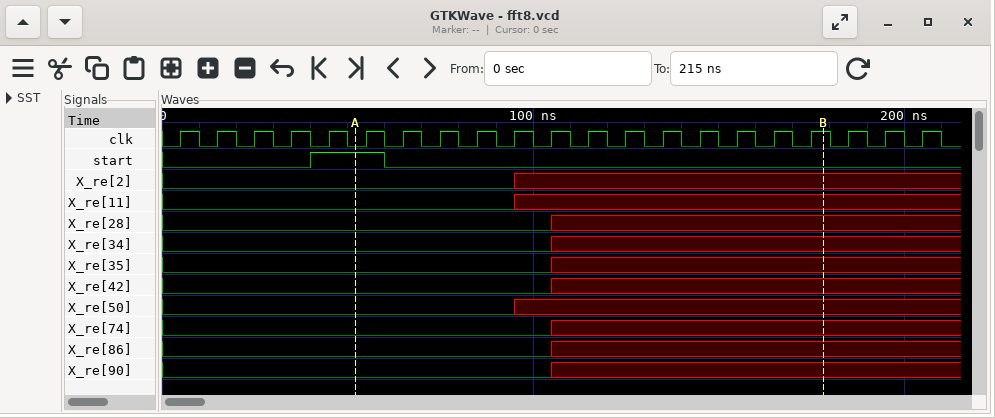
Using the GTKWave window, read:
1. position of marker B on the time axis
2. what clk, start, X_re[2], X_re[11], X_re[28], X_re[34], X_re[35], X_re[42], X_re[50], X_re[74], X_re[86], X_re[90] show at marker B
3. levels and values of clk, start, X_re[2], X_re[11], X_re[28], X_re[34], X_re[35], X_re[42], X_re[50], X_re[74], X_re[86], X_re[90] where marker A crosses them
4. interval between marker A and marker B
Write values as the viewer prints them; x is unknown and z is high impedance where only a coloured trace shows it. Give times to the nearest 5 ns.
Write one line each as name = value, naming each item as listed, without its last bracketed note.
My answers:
position of marker B on the time axis = 180 ns
what clk, start, X_re[2], X_re[11], X_re[28], X_re[34], X_re[35], X_re[42], X_re[50], X_re[74], X_re[86], X_re[90] show at marker B = clk=1, start=0, X_re[2]=x, X_re[11]=x, X_re[28]=x, X_re[34]=x, X_re[35]=x, X_re[42]=x, X_re[50]=x, X_re[74]=x, X_re[86]=x, X_re[90]=x
levels and values of clk, start, X_re[2], X_re[11], X_re[28], X_re[34], X_re[35], X_re[42], X_re[50], X_re[74], X_re[86], X_re[90] where marker A crosses them = clk=0, start=1, X_re[2]=0, X_re[11]=0, X_re[28]=0, X_re[34]=0, X_re[35]=0, X_re[42]=0, X_re[50]=0, X_re[74]=0, X_re[86]=0, X_re[90]=0
interval between marker A and marker B = 125 ns
